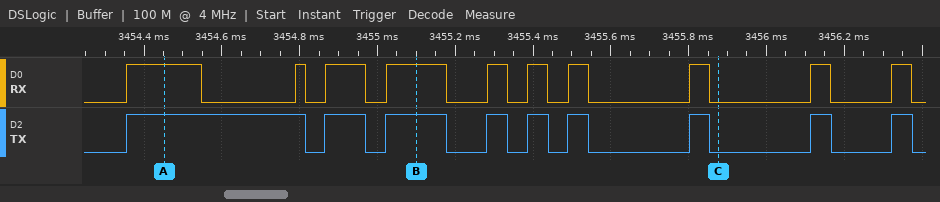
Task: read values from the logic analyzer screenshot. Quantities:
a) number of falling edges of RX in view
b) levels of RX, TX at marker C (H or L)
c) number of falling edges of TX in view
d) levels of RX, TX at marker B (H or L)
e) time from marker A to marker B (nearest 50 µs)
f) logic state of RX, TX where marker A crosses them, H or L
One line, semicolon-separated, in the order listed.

10; RX=L, TX=L; 9; RX=H, TX=H; 650 µs; RX=H, TX=H
